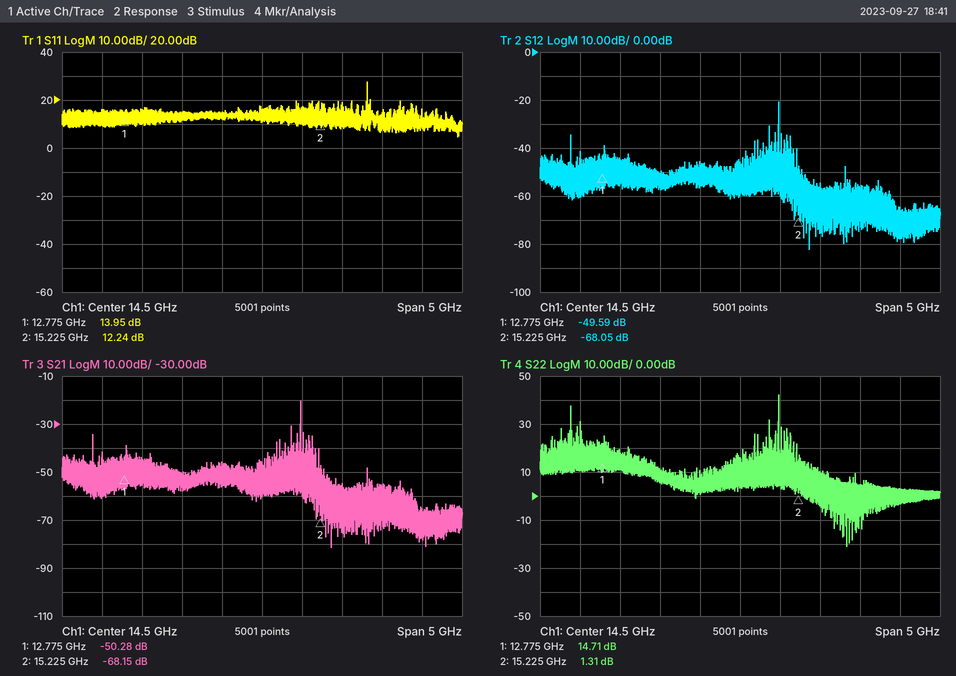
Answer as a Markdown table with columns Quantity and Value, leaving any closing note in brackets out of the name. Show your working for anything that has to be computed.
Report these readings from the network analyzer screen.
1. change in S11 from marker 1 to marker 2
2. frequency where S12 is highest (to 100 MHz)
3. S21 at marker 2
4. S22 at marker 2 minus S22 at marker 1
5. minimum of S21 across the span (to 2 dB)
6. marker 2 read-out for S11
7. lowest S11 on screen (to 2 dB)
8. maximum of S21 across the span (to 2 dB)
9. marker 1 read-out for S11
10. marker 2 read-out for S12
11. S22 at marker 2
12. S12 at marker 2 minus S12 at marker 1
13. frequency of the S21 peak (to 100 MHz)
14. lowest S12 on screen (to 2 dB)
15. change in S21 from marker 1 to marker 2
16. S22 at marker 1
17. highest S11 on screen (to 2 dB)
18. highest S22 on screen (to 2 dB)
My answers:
| Quantity | Value |
|---|---|
| change in S11 from marker 1 to marker 2 | 12.24 − (13.95) = -1.71 dB |
| frequency where S12 is highest | 15.0 GHz |
| S21 at marker 2 | -68.15 dB |
| S22 at marker 2 minus S22 at marker 1 | 1.31 − (14.71) = -13.40 dB |
| minimum of S21 across the span | -82 dB |
| marker 2 read-out for S11 | 12.24 dB |
| lowest S11 on screen | 4 dB |
| maximum of S21 across the span | -20 dB |
| marker 1 read-out for S11 | 13.95 dB |
| marker 2 read-out for S12 | -68.05 dB |
| S22 at marker 2 | 1.31 dB |
| S12 at marker 2 minus S12 at marker 1 | -68.05 − (-49.59) = -18.46 dB |
| frequency of the S21 peak | 15.0 GHz |
| lowest S12 on screen | -82 dB |
| change in S21 from marker 1 to marker 2 | -68.15 − (-50.28) = -17.87 dB |
| S22 at marker 1 | 14.71 dB |
| highest S11 on screen | 28 dB |
| highest S22 on screen | 42 dB |
